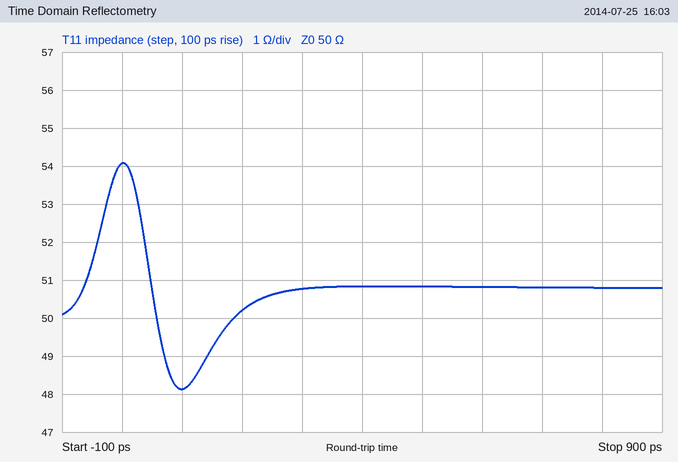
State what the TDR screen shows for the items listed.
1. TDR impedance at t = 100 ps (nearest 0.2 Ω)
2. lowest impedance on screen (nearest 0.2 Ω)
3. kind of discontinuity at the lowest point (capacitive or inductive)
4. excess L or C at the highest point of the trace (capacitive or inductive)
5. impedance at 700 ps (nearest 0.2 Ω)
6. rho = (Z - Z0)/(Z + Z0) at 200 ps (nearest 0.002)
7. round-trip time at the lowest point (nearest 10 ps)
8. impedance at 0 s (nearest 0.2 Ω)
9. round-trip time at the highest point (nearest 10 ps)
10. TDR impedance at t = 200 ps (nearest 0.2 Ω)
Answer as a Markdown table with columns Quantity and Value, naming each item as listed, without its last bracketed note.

| Quantity | Value |
|---|---|
| TDR impedance at t = 100 ps | 48.2 Ω |
| lowest impedance on screen | 48.2 Ω |
| kind of discontinuity at the lowest point | capacitive |
| excess L or C at the highest point of the trace | inductive |
| impedance at 700 ps | 50.8 Ω |
| rho = (Z - Z0)/(Z + Z0) at 200 ps | +0.002 |
| round-trip time at the lowest point | 100 ps |
| impedance at 0 s | 54.0 Ω |
| round-trip time at the highest point | 0 ps |
| TDR impedance at t = 200 ps | 50.2 Ω |
